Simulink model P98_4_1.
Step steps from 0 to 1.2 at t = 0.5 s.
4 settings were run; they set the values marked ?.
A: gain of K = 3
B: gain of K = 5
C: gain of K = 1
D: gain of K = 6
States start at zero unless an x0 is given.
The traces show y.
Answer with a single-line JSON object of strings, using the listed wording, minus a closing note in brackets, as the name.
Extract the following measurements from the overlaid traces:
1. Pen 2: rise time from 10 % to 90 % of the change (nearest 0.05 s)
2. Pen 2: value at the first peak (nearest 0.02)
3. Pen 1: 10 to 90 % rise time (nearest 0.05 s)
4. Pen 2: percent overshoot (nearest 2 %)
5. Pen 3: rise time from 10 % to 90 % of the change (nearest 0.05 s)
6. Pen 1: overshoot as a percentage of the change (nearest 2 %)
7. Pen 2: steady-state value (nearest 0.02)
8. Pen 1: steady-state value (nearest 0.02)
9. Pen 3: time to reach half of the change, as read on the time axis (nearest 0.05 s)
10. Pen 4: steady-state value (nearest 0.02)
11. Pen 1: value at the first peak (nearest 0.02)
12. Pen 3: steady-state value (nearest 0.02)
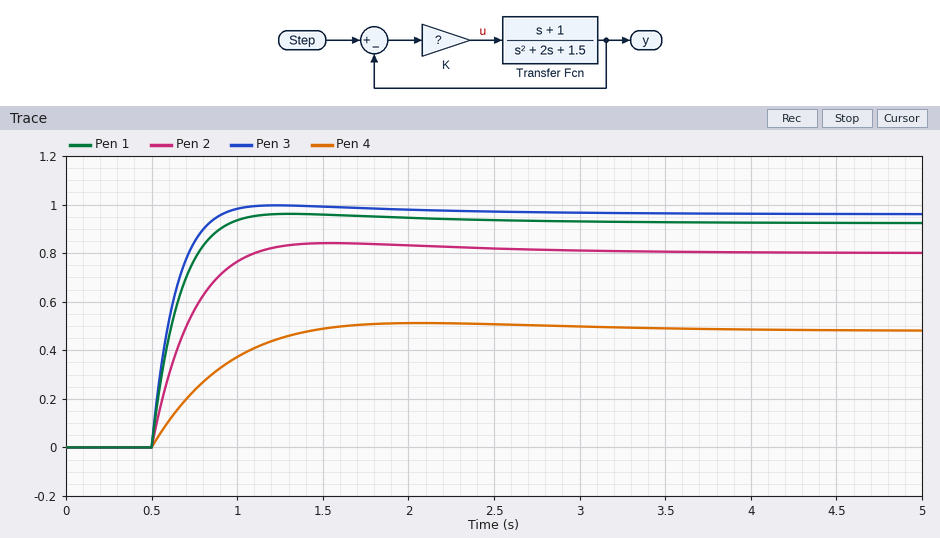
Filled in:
{"Pen 2: rise time from 10 % to 90 % of the change": "0.40 s", "Pen 2: value at the first peak": "0.84", "Pen 1: 10 to 90 % rise time": "0.30 s", "Pen 2: percent overshoot": "6 %", "Pen 3: rise time from 10 % to 90 % of the change": "0.25 s", "Pen 1: overshoot as a percentage of the change": "4 %", "Pen 2: steady-state value": "0.80", "Pen 1: steady-state value": "0.92", "Pen 3: time to reach half of the change, as read on the time axis": "0.60 s", "Pen 4: steady-state value": "0.48", "Pen 1: value at the first peak": "0.96", "Pen 3: steady-state value": "0.96"}
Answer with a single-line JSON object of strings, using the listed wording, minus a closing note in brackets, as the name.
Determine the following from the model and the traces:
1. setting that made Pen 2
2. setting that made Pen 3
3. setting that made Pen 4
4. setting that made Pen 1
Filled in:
{"setting that made Pen 2": "A", "setting that made Pen 3": "D", "setting that made Pen 4": "C", "setting that made Pen 1": "B"}
